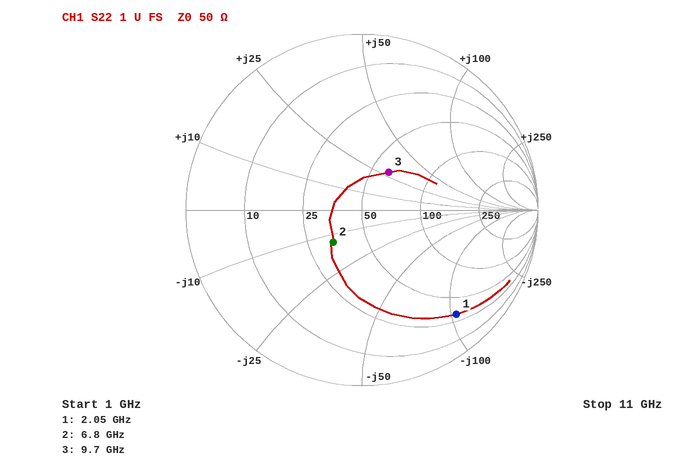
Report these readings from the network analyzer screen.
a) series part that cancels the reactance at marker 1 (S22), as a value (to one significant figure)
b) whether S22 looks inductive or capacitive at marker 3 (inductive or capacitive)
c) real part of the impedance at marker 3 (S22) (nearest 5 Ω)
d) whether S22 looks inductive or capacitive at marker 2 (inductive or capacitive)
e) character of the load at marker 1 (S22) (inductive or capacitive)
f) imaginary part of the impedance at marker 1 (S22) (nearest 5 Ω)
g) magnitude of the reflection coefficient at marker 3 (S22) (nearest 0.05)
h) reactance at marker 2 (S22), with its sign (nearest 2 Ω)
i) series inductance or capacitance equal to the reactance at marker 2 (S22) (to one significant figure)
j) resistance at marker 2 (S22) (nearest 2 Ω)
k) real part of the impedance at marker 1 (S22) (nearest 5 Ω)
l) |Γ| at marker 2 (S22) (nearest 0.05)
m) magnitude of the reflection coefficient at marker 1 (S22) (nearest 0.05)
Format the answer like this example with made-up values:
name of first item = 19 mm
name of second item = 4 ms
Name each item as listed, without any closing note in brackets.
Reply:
series part that cancels the reactance at marker 1 (S22), as a value = 8 nH
whether S22 looks inductive or capacitive at marker 3 = inductive
real part of the impedance at marker 3 (S22) = 60 Ω
whether S22 looks inductive or capacitive at marker 2 = capacitive
character of the load at marker 1 (S22) = capacitive
imaginary part of the impedance at marker 1 (S22) = -105 Ω
magnitude of the reflection coefficient at marker 3 (S22) = 0.25
reactance at marker 2 (S22), with its sign = -14 Ω
series inductance or capacitance equal to the reactance at marker 2 (S22) = 2 pF
resistance at marker 2 (S22) = 34 Ω
real part of the impedance at marker 1 (S22) = 30 Ω
|Γ| at marker 2 (S22) = 0.25
magnitude of the reflection coefficient at marker 1 (S22) = 0.80
